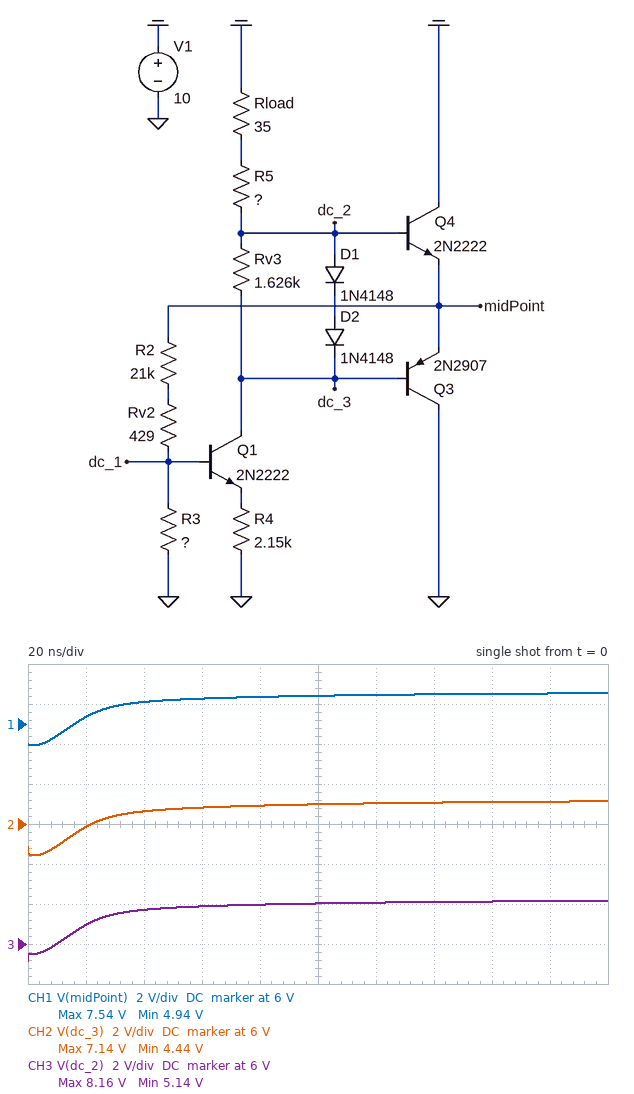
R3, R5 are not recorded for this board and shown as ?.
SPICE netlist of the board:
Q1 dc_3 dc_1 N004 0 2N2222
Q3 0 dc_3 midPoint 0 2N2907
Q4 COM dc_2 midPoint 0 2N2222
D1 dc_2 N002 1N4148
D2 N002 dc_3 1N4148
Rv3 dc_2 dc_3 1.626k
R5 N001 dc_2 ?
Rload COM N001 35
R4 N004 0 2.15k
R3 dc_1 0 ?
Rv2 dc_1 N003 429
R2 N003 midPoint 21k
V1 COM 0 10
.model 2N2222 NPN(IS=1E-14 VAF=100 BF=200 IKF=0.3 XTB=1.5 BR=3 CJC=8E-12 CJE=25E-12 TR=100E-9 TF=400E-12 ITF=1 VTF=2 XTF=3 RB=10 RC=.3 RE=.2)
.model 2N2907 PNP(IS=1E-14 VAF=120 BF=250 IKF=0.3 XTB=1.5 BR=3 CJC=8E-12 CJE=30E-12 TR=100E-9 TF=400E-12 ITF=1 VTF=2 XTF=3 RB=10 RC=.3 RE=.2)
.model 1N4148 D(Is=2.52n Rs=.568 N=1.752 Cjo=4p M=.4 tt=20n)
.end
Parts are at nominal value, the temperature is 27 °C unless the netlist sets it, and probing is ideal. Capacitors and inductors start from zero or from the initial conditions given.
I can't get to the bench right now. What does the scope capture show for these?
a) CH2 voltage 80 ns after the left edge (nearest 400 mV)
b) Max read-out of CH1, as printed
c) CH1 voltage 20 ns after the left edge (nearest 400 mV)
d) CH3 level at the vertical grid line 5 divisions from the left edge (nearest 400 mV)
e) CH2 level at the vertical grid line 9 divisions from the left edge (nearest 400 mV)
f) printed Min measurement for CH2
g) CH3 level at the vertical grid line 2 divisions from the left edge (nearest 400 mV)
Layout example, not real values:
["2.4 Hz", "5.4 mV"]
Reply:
["6.8 V", "7.54 V", "6.4 V", "8.0 V", "7.2 V", "4.44 V", "7.6 V"]
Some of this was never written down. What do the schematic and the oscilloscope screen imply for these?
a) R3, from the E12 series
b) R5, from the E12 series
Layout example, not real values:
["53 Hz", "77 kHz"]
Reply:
["10 kΩ", "2.2 kΩ"]
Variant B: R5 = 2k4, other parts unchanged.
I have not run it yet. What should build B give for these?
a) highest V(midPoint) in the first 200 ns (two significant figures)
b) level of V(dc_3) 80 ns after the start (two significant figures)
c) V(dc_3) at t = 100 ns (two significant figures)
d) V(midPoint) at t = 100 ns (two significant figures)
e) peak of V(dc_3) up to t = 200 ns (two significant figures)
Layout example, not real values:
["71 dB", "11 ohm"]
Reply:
["7.4 V", "6.8 V", "6.9 V", "7.3 V", "7.0 V"]
